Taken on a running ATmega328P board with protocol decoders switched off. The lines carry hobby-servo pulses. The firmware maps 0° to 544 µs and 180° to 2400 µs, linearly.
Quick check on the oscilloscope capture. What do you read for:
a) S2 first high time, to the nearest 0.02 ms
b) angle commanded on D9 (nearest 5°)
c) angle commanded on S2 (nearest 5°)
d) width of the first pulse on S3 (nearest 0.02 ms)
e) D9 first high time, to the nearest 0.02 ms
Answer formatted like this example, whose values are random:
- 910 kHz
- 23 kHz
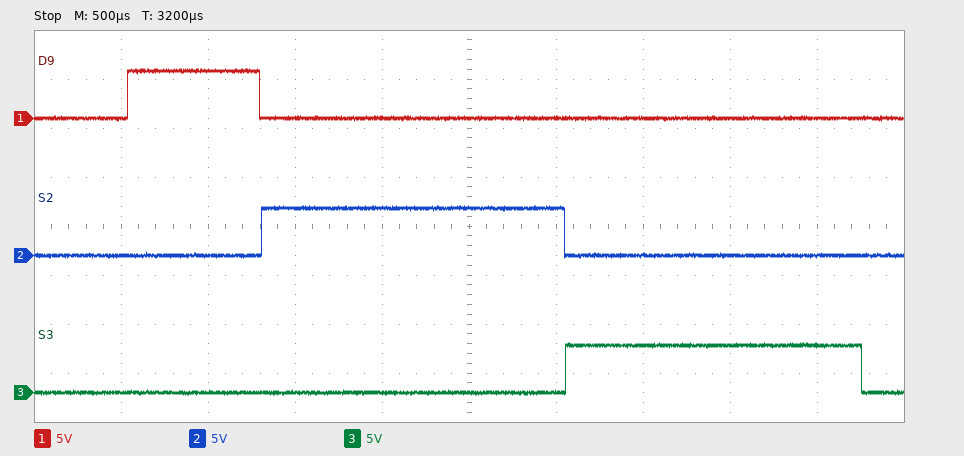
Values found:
- 1.74 ms
- 20°
- 115°
- 1.70 ms
- 0.76 ms
